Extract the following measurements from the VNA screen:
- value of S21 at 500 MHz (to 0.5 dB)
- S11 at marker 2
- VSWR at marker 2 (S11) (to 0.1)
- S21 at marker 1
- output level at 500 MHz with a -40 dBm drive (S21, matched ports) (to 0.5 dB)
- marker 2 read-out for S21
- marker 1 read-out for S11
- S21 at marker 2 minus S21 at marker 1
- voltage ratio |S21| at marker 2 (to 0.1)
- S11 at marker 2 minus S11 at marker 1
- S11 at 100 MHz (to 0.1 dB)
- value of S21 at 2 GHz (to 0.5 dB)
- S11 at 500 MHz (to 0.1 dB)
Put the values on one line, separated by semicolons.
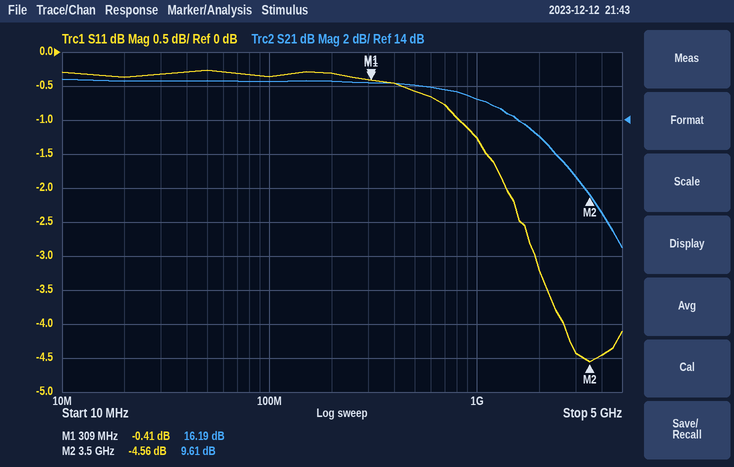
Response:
16.0 dB; -4.56 dB; 3.9; 16.19 dB; -24.0 dBm; 9.61 dB; -0.41 dB; -6.58 dB; 3.0; -4.15 dB; -0.4 dB; 13.0 dB; -0.6 dB
